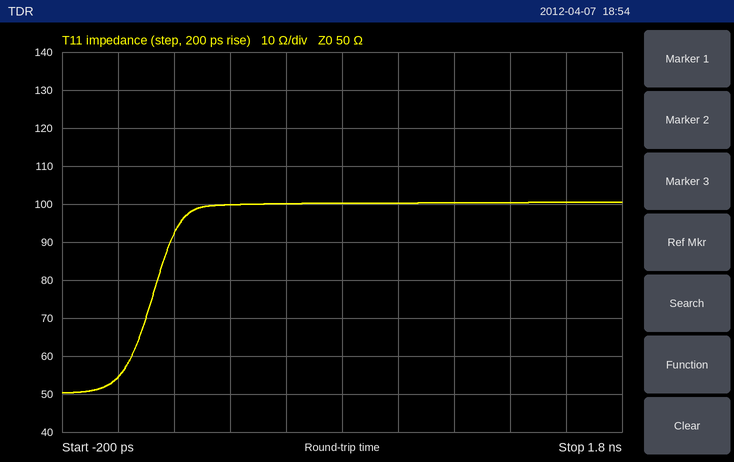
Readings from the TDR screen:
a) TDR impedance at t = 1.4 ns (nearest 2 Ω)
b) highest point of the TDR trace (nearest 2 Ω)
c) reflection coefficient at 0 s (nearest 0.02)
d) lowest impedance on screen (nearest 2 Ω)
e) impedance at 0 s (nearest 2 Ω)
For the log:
100 Ω
100 Ω
+0.04
50 Ω
54 Ω
